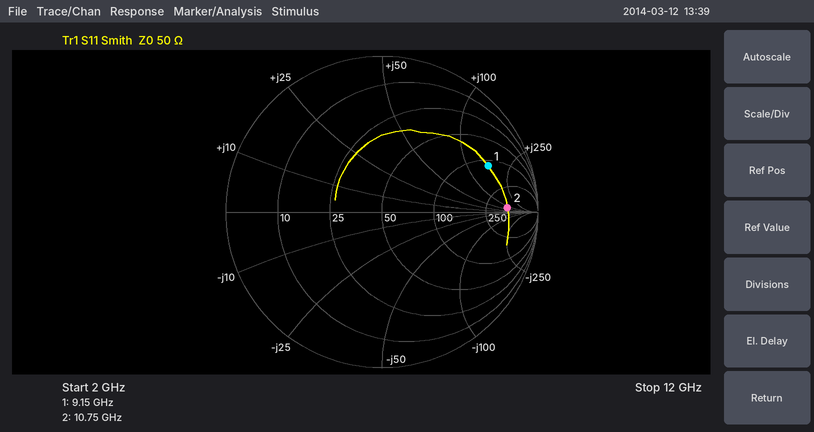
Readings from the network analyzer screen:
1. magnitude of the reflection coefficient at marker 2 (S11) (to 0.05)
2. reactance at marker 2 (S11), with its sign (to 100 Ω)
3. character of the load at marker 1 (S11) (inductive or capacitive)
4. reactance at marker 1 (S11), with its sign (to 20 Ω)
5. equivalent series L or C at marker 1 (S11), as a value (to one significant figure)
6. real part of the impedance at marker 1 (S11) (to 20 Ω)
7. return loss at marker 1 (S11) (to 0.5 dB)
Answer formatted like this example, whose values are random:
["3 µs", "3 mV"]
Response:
["0.80", "+100 Ω", "inductive", "+160 Ω", "3 nH", "120 Ω", "2.5 dB"]
